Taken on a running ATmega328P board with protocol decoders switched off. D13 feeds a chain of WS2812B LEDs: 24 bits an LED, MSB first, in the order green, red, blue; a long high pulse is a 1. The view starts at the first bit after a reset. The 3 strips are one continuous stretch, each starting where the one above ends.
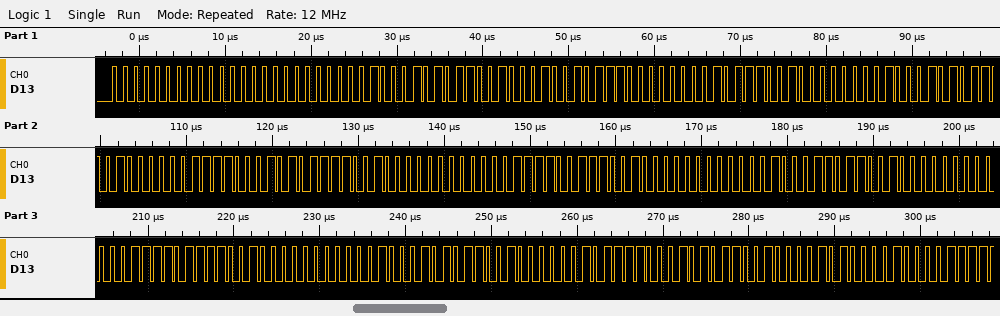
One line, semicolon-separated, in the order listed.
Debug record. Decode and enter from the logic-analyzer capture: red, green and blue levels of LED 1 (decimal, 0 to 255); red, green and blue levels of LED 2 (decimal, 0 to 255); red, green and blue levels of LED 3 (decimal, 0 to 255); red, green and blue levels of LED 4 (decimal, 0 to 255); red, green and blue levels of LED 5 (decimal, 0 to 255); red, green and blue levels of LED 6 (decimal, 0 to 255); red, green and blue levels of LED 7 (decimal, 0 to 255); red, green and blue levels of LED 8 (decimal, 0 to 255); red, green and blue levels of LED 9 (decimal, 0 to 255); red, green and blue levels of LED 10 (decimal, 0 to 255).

0, 0, 0; 200, 138, 151; 185, 0, 0; 200, 138, 30; 200, 43, 0; 200, 121, 0; 200, 70, 0; 200, 123, 0; 200, 138, 23; 200, 138, 80
